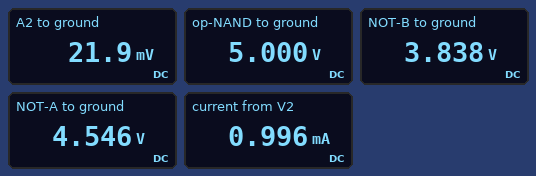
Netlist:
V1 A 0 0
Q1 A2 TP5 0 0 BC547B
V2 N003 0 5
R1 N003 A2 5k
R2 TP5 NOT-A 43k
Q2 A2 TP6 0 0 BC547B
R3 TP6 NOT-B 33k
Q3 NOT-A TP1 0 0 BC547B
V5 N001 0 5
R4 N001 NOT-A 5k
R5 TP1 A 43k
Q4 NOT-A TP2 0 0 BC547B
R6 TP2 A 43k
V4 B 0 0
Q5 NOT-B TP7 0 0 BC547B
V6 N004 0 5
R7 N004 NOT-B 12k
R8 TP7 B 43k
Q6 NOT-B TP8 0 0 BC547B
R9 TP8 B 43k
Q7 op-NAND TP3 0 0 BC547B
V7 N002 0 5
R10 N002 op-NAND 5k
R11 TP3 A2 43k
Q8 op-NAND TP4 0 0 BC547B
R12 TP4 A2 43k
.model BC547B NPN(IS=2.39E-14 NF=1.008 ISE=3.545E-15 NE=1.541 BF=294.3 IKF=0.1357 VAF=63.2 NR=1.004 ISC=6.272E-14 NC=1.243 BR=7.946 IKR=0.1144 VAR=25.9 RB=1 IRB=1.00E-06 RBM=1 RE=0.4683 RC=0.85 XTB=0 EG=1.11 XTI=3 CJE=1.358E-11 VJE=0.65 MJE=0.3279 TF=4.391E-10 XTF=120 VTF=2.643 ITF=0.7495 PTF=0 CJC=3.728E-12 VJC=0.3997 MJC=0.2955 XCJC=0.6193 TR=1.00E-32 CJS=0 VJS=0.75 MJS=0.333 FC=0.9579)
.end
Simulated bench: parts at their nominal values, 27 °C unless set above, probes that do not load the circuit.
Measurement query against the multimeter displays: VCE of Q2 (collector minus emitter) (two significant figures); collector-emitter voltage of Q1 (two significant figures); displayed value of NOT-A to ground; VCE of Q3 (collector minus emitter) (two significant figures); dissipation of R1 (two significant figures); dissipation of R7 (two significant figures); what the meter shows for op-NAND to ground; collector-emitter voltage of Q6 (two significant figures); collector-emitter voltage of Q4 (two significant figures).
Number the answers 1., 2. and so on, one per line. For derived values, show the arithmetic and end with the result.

1. 21.9 mV = 22 mV
2. 21.9 mV = 22 mV
3. 4.546 V
4. 4.546 V = 4.5 V
5. (5 V - 21.9 mV)^2 / 5 kΩ = 5.0 mW
6. (5 V - 3.838 V)^2 / 12 kΩ = 110 µW
7. 5.000 V
8. 3.838 V = 3.8 V
9. 4.546 V = 4.5 V
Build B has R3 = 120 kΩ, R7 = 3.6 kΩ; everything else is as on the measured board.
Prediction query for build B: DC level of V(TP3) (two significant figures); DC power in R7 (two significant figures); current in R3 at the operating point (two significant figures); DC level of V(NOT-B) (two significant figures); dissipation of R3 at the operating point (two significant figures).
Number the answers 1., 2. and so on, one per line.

1. 27 mV
2. 4.5 µW
3. 35 µA
4. 4.9 V
5. 150 µW
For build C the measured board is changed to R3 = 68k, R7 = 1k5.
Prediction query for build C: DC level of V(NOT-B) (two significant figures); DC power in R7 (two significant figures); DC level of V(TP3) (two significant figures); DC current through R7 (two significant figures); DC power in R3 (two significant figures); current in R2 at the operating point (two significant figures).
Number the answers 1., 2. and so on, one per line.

1. 4.9 V
2. 5.9 µW
3. 24 mV
4. 63 µA
5. 270 µW
6. 91 µA
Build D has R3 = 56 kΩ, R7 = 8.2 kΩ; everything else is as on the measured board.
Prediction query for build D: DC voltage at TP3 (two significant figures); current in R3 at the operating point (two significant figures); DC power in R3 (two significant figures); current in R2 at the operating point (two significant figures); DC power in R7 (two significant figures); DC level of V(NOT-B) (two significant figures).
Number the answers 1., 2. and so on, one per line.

1. 24 mV
2. 68 µA
3. 260 µW
4. 91 µA
5. 38 µW
6. 4.4 V
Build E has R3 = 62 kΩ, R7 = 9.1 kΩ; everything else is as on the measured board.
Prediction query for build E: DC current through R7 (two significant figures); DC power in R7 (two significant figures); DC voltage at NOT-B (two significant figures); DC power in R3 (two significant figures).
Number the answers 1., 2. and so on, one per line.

1. 61 µA
2. 34 µW
3. 4.4 V
4. 230 µW
